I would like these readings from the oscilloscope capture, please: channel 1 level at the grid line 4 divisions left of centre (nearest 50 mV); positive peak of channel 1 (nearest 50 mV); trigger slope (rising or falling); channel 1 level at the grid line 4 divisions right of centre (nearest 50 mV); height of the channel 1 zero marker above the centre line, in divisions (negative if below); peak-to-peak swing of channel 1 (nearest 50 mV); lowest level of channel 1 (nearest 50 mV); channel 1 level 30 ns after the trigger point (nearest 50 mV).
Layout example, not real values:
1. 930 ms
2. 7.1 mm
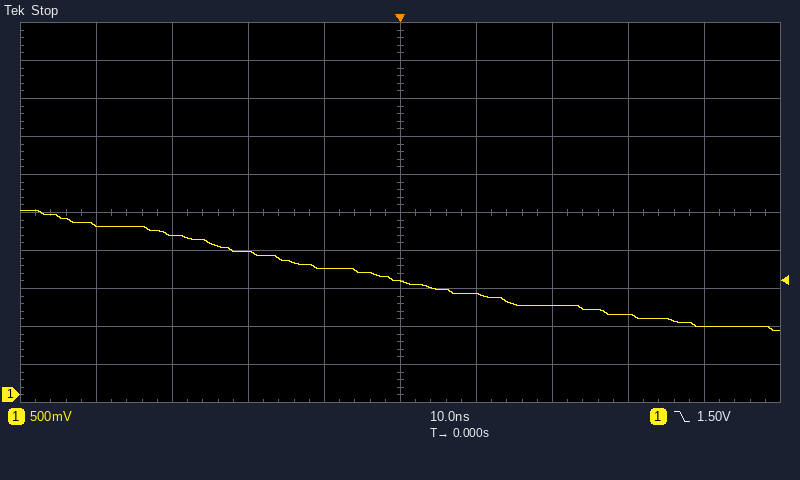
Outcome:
1. 2.25 V
2. 2.45 V
3. falling
4. 900 mV
5. -4.8 div
6. 1.60 V
7. 850 mV
8. 1.05 V
